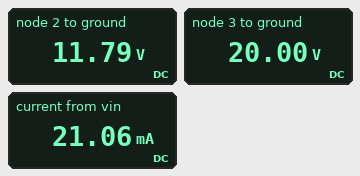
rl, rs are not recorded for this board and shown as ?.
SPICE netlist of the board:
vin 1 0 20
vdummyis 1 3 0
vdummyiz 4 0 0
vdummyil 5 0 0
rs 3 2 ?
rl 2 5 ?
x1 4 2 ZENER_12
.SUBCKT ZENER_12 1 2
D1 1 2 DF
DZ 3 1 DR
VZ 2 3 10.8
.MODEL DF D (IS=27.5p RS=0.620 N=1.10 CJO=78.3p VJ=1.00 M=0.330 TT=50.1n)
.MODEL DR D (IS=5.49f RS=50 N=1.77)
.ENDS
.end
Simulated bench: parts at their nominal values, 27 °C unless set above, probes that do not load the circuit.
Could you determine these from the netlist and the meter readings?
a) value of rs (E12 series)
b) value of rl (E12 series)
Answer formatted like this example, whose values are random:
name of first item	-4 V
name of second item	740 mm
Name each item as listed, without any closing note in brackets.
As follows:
value of rs	390 Ω
value of rl	560 Ω
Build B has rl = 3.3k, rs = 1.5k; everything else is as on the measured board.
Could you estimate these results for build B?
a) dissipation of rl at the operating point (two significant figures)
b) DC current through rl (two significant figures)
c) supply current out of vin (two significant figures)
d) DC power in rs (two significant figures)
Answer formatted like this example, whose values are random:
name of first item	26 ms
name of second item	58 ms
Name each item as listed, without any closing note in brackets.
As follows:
dissipation of rl at the operating point	44 mW
DC current through rl	3.7 mA
supply current out of vin	5.3 mA
DC power in rs	42 mW
